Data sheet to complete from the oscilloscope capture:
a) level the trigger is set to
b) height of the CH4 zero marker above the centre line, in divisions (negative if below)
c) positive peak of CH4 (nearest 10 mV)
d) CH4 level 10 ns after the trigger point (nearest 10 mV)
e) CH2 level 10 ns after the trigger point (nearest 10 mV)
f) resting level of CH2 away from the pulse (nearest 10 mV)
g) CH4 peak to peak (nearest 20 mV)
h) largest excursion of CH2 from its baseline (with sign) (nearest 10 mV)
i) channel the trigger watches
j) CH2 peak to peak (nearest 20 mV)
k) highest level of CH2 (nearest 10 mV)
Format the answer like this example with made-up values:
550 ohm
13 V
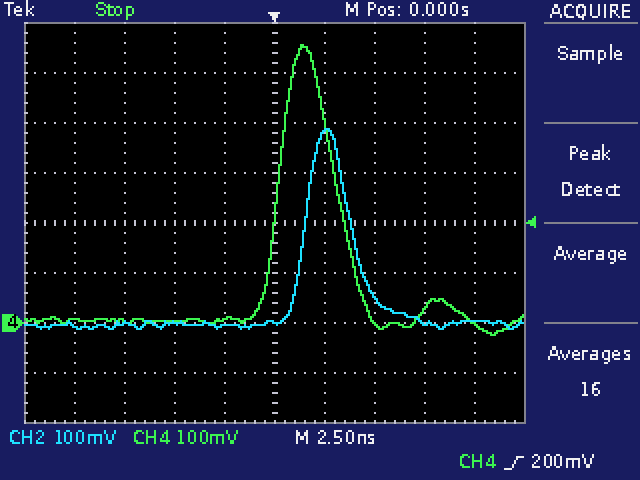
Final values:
200 mV
-2.0 div
560 mV
0 mV
0 mV
0 mV
580 mV
+390 mV
CH4
400 mV
390 mV
